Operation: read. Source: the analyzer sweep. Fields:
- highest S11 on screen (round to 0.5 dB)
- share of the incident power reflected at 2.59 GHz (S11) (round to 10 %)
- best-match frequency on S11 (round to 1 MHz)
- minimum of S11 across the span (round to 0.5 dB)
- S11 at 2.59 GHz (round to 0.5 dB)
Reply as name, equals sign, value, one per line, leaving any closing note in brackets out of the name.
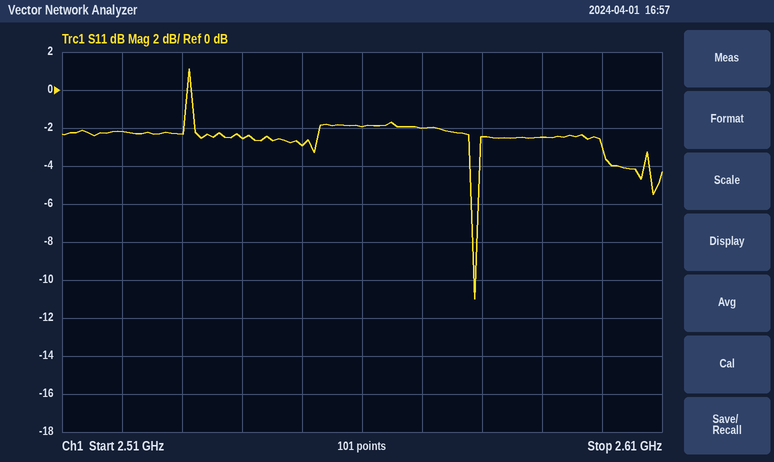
highest S11 on screen = 1.0 dB
share of the incident power reflected at 2.59 GHz (S11) = 60 %
best-match frequency on S11 = 2.579 GHz
minimum of S11 across the span = -11.0 dB
S11 at 2.59 GHz = -2.5 dB
